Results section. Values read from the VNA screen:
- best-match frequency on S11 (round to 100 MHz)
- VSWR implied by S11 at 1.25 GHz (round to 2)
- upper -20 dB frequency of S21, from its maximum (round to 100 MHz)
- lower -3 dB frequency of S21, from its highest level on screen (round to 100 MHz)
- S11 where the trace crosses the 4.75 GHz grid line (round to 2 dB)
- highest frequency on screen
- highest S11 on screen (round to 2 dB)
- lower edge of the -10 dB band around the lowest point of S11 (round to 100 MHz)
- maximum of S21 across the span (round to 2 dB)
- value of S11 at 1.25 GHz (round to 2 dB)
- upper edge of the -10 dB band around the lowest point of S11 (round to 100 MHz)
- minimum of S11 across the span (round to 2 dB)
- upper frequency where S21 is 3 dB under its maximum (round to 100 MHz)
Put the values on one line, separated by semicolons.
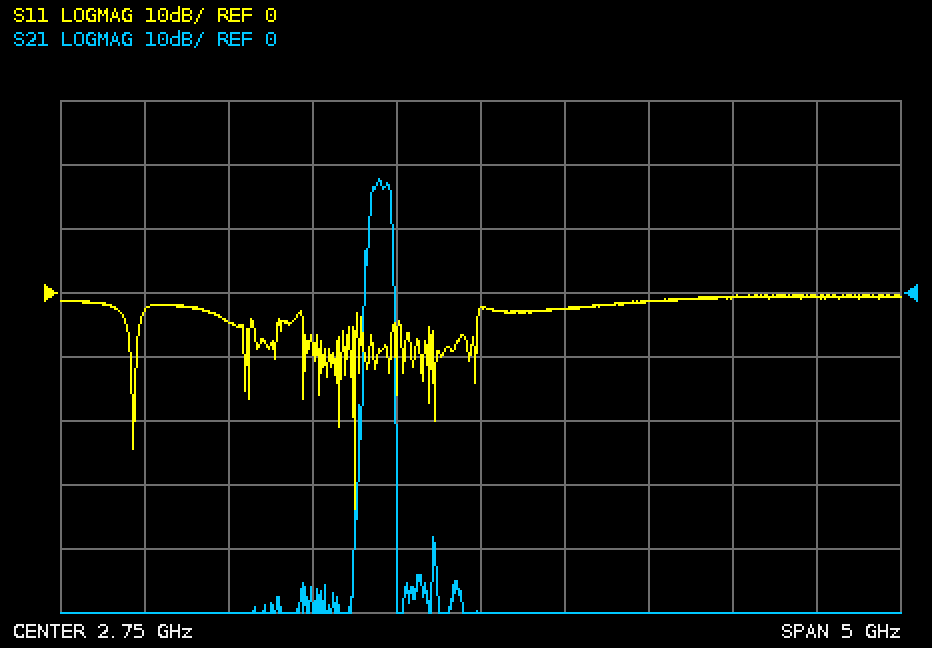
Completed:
2.0 GHz; 4; 2.2 GHz; 2.1 GHz; 0 dB; 5.25 GHz; 0 dB; 2.0 GHz; 18 dB; -4 dB; 2.0 GHz; -34 dB; 2.2 GHz
